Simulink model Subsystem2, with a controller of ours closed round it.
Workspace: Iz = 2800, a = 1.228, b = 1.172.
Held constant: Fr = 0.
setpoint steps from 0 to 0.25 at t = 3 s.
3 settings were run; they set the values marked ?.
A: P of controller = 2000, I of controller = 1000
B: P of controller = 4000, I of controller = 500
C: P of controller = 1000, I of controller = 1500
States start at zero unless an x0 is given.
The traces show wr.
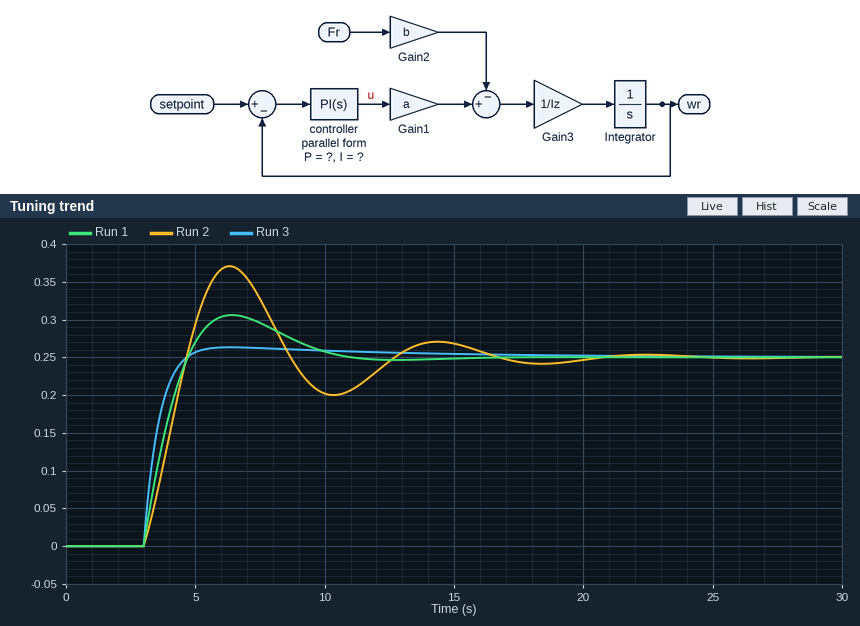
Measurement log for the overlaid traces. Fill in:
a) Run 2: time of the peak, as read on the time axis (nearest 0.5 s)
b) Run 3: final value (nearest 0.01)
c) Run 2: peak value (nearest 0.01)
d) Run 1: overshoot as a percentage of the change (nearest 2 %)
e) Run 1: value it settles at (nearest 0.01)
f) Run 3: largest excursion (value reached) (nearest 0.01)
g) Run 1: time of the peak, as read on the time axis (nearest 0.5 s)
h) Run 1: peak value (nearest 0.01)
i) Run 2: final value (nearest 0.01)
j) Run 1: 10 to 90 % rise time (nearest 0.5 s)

6.5 s
0.25
0.37
22 %
0.25
0.26
6.5 s
0.31
0.25
1.5 s
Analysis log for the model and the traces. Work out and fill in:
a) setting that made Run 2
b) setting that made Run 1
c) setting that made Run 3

C
A
B
